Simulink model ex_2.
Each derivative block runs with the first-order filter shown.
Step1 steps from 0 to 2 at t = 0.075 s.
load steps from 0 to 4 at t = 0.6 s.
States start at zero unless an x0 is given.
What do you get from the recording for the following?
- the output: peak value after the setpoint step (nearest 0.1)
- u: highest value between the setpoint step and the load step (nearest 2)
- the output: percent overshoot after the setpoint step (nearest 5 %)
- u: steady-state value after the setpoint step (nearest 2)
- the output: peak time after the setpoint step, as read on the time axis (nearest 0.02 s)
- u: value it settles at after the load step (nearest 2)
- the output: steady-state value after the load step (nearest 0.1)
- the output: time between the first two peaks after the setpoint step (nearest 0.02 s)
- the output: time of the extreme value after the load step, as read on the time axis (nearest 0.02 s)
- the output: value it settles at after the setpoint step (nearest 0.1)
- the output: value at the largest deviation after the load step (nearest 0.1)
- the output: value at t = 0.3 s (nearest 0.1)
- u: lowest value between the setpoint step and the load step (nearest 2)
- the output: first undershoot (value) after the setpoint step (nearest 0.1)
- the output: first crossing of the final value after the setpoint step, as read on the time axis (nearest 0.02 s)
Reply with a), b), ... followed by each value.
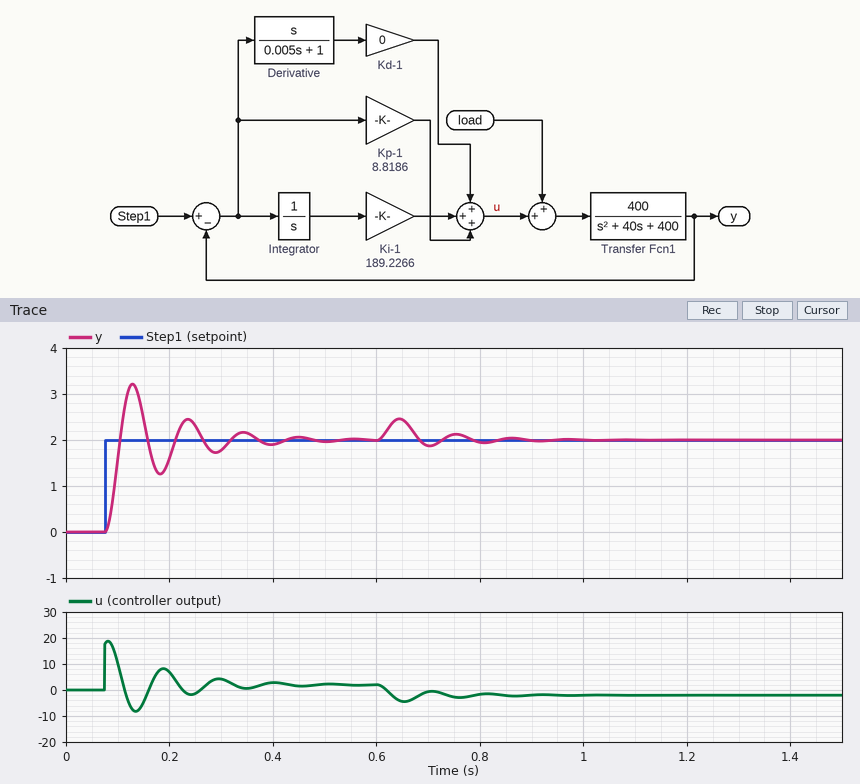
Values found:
a) 3.2
b) 18
c) 60 %
d) 2
e) 0.12 s
f) -2
g) 2.0
h) 0.10 s
i) 0.64 s
j) 2.0
k) 2.5
l) 1.8
m) -8
n) 1.3
o) 0.10 s
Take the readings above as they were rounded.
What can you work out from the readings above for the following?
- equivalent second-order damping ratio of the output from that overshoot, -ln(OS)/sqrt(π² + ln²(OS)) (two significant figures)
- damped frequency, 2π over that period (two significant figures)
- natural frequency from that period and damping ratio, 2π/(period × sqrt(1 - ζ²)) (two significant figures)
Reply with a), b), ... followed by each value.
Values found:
a) 0.16
b) 63 rad/s
c) 64 rad/s
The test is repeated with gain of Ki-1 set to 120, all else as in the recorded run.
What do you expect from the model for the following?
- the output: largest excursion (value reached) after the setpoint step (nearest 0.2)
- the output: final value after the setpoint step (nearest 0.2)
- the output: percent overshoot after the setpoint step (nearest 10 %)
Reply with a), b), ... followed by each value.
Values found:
a) 3.0
b) 2.0
c) 50 %
